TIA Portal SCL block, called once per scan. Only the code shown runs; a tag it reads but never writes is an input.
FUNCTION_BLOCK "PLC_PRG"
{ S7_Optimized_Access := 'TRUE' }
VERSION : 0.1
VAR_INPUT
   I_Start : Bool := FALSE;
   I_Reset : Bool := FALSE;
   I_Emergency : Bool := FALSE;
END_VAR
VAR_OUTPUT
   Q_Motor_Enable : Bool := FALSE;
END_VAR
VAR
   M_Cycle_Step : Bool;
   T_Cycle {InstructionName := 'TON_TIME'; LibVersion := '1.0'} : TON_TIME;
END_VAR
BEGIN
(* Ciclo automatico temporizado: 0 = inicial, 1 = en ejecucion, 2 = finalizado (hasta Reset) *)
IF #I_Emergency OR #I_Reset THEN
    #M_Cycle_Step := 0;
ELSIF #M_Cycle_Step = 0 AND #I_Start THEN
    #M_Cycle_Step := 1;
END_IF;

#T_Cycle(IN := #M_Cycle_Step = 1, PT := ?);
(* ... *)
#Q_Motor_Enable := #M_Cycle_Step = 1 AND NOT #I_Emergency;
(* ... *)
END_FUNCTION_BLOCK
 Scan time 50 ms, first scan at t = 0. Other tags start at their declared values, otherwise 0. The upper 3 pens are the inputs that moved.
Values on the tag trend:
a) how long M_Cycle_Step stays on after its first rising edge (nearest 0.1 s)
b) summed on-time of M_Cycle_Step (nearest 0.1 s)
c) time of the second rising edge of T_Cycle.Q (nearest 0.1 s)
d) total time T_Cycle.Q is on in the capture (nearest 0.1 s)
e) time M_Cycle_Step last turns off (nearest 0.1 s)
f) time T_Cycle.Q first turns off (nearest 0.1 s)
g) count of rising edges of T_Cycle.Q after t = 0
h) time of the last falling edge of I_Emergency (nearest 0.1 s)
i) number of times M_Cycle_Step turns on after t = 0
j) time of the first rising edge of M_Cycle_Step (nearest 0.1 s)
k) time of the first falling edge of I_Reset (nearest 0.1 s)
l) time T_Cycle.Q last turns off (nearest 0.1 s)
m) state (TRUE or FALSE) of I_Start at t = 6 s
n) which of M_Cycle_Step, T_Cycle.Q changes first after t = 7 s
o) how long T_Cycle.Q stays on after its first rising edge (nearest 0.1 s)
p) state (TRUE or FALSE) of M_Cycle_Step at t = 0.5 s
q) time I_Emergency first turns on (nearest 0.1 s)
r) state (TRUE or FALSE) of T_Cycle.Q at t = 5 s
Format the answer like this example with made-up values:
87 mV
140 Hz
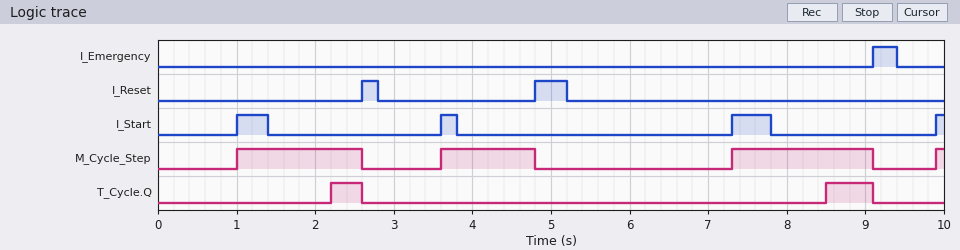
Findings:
1.6 s
4.7 s
8.5 s
1.0 s
9.1 s
2.6 s
2
9.4 s
4
1.0 s
2.8 s
9.1 s
FALSE
M_Cycle_Step
0.4 s
FALSE
9.1 s
FALSE
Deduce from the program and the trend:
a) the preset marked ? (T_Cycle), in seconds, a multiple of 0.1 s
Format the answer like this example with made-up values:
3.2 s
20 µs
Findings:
1.2 s
